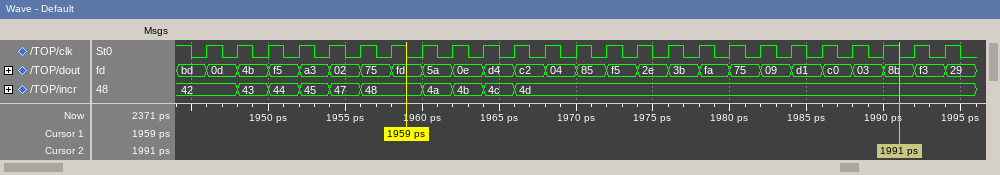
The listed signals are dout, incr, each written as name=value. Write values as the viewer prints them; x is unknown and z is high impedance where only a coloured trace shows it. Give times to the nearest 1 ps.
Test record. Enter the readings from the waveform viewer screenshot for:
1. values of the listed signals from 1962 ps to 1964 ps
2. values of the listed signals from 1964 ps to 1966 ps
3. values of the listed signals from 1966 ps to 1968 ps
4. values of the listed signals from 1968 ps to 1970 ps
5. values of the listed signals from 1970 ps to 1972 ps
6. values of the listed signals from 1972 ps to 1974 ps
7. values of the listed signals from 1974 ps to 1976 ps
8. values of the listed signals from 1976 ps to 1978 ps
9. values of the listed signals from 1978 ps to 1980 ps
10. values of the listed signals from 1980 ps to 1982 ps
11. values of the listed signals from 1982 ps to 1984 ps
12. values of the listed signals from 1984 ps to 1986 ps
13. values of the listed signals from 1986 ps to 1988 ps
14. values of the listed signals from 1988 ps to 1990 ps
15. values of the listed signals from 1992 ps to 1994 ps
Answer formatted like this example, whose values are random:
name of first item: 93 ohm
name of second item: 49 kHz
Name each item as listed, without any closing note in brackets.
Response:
values of the listed signals from 1962 ps to 1964 ps: dout=0e, incr=4b
values of the listed signals from 1964 ps to 1966 ps: dout=d4, incr=4c
values of the listed signals from 1966 ps to 1968 ps: dout=c2, incr=4d
values of the listed signals from 1968 ps to 1970 ps: dout=04, incr=4d
values of the listed signals from 1970 ps to 1972 ps: dout=85, incr=4d
values of the listed signals from 1972 ps to 1974 ps: dout=f5, incr=4d
values of the listed signals from 1974 ps to 1976 ps: dout=2e, incr=4d
values of the listed signals from 1976 ps to 1978 ps: dout=3b, incr=4d
values of the listed signals from 1978 ps to 1980 ps: dout=fa, incr=4d
values of the listed signals from 1980 ps to 1982 ps: dout=75, incr=4d
values of the listed signals from 1982 ps to 1984 ps: dout=09, incr=4d
values of the listed signals from 1984 ps to 1986 ps: dout=d1, incr=4d
values of the listed signals from 1986 ps to 1988 ps: dout=c0, incr=4d
values of the listed signals from 1988 ps to 1990 ps: dout=03, incr=4d
values of the listed signals from 1992 ps to 1994 ps: dout=f3, incr=4d
